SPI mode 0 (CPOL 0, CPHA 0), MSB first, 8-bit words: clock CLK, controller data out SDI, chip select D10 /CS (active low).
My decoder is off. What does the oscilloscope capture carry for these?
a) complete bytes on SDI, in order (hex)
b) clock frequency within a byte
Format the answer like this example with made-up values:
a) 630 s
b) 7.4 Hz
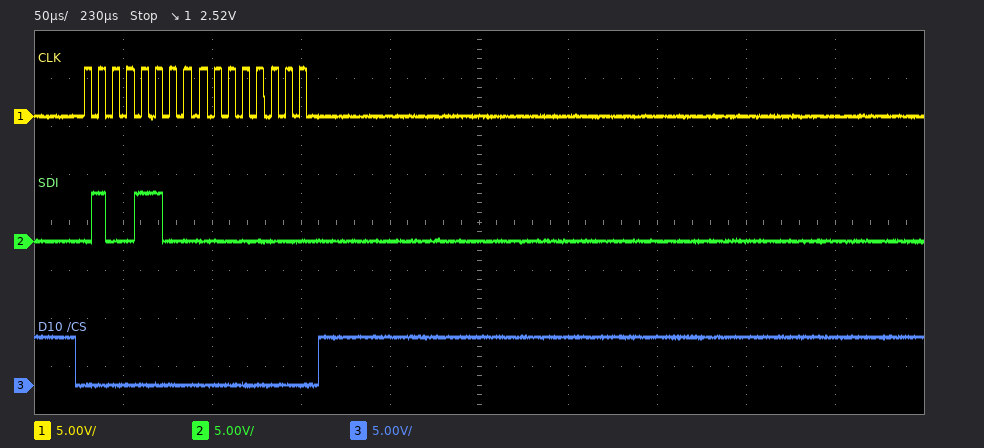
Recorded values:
a) 4C 00
b) 125 kHz
